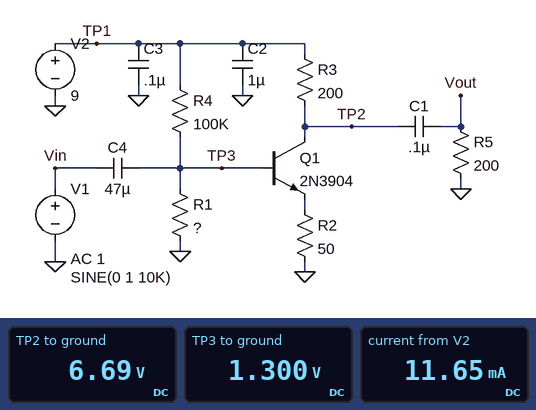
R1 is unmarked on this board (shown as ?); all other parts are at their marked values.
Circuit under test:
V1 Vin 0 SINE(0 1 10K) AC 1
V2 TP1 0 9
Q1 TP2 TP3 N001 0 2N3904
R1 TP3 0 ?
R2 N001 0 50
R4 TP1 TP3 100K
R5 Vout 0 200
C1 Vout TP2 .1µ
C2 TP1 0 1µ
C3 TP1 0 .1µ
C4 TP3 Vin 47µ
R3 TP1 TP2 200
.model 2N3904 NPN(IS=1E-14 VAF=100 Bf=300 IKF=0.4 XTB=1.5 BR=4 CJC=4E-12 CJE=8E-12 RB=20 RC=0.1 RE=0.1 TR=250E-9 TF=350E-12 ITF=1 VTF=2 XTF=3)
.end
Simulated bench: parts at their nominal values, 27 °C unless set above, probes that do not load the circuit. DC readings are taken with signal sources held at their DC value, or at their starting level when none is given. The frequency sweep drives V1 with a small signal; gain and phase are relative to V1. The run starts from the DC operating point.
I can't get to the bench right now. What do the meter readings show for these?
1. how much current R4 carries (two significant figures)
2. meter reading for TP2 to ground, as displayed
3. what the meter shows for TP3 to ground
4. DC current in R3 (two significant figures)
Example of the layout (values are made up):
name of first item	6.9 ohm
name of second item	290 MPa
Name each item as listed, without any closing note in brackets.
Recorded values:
how much current R4 carries	77 µA
meter reading for TP2 to ground, as displayed	6.69 V
what the meter shows for TP3 to ground	1.300 V
DC current in R3	12 mA
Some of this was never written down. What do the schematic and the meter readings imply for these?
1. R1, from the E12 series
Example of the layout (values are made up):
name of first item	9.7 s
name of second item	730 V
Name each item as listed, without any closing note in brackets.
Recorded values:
R1, from the E12 series	33 kΩ
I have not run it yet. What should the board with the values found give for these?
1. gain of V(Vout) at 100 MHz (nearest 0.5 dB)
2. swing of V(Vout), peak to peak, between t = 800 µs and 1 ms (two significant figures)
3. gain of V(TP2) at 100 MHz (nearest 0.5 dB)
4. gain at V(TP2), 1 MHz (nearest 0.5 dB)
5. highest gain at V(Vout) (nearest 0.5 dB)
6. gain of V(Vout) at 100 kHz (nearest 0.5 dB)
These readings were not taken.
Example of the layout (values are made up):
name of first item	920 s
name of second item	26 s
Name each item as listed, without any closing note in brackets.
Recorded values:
gain of V(Vout) at 100 MHz	5.0 dB
swing of V(Vout), peak to peak, between t = 800 µs and 1 ms	3.2 V
gain of V(TP2) at 100 MHz	5.0 dB
gain at V(TP2), 1 MHz	5.5 dB
highest gain at V(Vout)	5.5 dB
gain of V(Vout) at 100 kHz	5.5 dB
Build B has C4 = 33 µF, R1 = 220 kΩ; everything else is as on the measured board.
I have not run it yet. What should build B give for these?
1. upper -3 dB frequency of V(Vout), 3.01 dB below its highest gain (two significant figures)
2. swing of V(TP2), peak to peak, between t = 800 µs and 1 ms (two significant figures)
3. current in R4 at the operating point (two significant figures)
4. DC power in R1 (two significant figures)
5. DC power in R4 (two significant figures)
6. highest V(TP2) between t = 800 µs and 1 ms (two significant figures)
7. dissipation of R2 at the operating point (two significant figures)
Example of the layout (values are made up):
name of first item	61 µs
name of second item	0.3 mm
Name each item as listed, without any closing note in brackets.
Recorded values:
upper -3 dB frequency of V(Vout), 3.01 dB below its highest gain	280 MHz
swing of V(TP2), peak to peak, between t = 800 µs and 1 ms	4.5 V
current in R4 at the operating point	73 µA
DC power in R1	13 µW
DC power in R4	530 µW
highest V(TP2) between t = 800 µs and 1 ms	7.3 V
dissipation of R2 at the operating point	19 mW
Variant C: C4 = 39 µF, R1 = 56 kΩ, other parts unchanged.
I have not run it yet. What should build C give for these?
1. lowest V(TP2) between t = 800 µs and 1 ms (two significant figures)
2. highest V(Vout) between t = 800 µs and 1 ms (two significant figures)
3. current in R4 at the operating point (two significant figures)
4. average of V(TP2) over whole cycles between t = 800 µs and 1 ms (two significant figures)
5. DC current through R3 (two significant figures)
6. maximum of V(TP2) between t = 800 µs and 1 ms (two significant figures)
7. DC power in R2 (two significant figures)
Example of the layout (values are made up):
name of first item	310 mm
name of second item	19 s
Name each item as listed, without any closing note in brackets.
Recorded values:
lowest V(TP2) between t = 800 µs and 1 ms	3.7 V
highest V(Vout) between t = 800 µs and 1 ms	1.6 V
current in R4 at the operating point	75 µA
average of V(TP2) over whole cycles between t = 800 µs and 1 ms	5.9 V
DC current through R3	15 mA
maximum of V(TP2) between t = 800 µs and 1 ms	7.9 V
DC power in R2	11 mW
